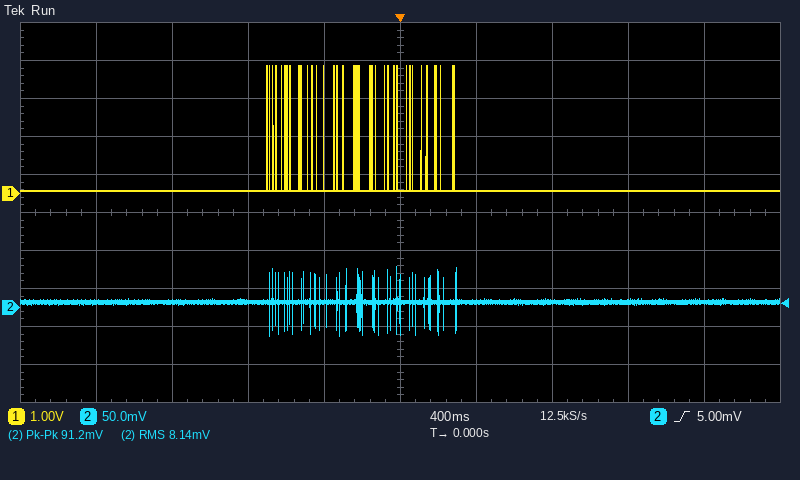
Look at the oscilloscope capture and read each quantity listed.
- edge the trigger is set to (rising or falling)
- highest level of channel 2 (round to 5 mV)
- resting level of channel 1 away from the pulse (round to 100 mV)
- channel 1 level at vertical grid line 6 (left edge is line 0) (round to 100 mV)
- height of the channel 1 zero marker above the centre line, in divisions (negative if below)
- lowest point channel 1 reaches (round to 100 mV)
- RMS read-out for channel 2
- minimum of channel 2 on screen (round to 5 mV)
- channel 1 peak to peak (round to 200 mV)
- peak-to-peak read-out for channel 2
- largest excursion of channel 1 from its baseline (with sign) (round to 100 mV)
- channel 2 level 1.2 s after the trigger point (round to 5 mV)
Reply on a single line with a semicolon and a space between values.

rising; 55 mV; 100 mV; 100 mV; +0.5 div; 100 mV; 8.14 mV; -35 mV; 3.2 V; 91.2 mV; +3.3 V; 10 mV
